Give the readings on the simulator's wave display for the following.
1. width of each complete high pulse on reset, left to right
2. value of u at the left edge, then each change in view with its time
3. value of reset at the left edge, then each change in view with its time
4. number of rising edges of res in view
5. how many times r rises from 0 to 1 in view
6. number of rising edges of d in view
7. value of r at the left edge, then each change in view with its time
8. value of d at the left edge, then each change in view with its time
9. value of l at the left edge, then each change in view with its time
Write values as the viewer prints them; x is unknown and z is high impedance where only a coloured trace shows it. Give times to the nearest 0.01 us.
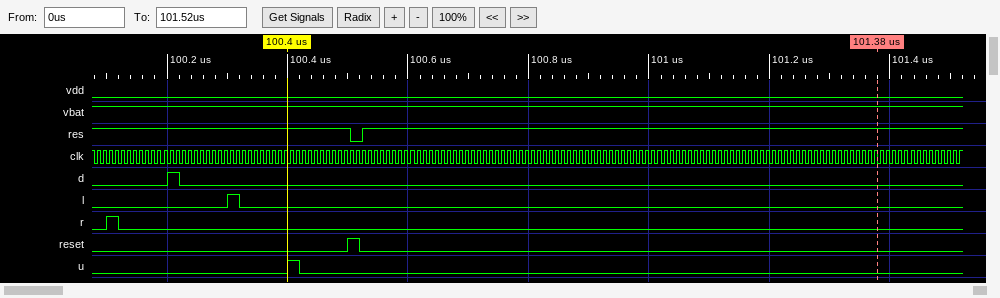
0.02 us
0, 1 at 100.4 us, 0 at 100.42 us
0, 1 at 100.5 us, 0 at 100.52 us
1
1
1
0, 1 at 100.1 us, 0 at 100.12 us
0, 1 at 100.2 us, 0 at 100.22 us
0, 1 at 100.3 us, 0 at 100.32 us
